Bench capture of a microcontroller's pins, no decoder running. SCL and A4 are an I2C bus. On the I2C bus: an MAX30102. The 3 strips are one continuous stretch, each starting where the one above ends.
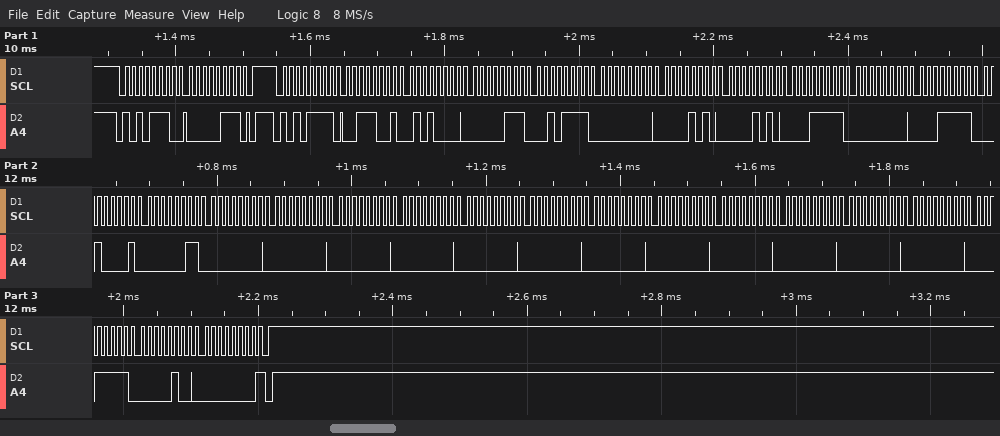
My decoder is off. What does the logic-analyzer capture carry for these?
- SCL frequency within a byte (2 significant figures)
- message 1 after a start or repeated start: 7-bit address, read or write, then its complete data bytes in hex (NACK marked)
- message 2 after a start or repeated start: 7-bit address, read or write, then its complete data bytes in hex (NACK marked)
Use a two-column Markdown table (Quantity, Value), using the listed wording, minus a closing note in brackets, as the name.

| Quantity | Value |
|---|---|
| SCL frequency within a byte | 100 kHz |
| message 1 after a start or repeated start: 7-bit address, read or write, then its complete data bytes in hex | 0x57 write: 07 |
| message 2 after a start or repeated start: 7-bit address, read or write, then its complete data bytes in hex | 0x57 read: 39 50 07 2F 00 0A 0A 1F 00 1F 21 03 00 00 00 00 00 00 00 00 00 00 00 00 1F 04 00 NACK |
